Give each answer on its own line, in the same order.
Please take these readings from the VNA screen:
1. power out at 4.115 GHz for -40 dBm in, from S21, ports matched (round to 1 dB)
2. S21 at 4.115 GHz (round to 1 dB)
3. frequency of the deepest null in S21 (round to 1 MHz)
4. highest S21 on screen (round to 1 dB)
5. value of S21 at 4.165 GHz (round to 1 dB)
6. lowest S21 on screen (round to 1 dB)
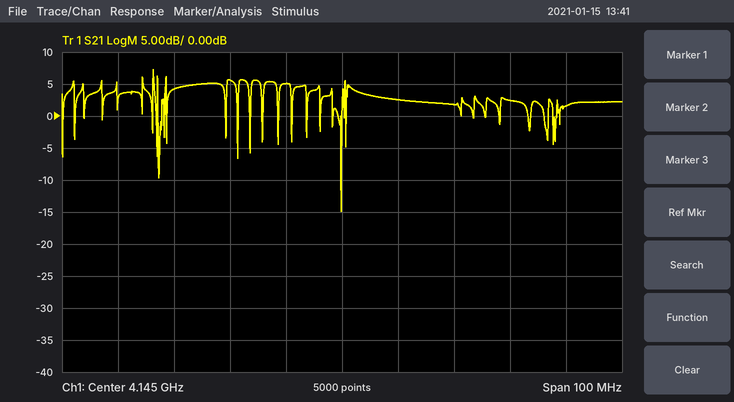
-36 dBm
4 dB
4.145 GHz
7 dB
2 dB
-15 dB
